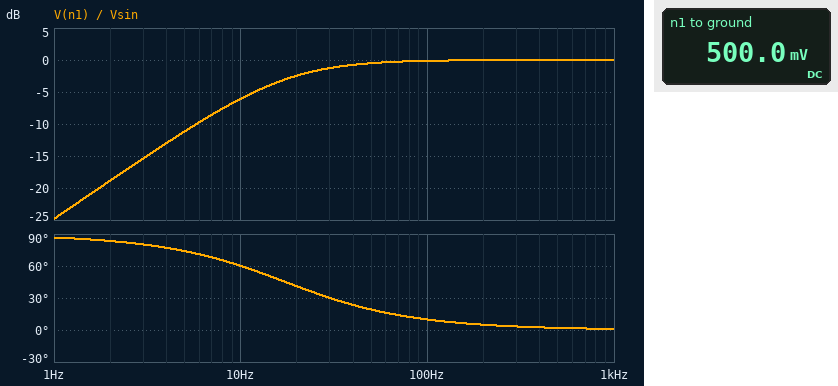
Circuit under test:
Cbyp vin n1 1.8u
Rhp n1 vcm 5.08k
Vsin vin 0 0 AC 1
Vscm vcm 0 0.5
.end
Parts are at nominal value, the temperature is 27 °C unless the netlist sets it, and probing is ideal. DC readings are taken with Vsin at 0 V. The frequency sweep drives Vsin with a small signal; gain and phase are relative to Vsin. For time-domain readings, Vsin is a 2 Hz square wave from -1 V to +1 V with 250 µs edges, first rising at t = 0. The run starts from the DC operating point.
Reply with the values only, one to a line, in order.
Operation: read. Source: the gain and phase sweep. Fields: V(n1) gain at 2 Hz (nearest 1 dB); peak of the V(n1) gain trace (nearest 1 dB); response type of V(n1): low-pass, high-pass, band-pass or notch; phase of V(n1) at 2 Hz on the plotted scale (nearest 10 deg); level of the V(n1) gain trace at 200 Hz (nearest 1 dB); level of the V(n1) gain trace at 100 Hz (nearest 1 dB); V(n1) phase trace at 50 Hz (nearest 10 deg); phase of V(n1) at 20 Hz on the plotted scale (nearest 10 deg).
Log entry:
-19 dB
0 dB
high-pass
80 deg
0 dB
0 dB
20 deg
40 deg
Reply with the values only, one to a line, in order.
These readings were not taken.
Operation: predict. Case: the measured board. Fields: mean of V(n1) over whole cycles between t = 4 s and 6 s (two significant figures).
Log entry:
500 mV
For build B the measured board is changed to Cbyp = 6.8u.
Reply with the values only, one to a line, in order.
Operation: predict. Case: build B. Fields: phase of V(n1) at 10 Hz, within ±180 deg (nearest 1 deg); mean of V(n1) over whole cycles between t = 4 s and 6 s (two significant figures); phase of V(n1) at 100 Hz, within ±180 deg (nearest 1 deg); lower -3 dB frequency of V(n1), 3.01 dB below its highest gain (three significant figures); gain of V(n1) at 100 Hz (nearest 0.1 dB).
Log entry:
25 deg
500 mV
3 deg
4.61 Hz
0 dB
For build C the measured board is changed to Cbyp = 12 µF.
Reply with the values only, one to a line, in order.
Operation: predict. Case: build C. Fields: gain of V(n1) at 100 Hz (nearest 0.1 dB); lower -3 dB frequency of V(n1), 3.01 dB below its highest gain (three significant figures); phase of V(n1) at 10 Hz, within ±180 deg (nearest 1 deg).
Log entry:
0 dB
2.61 Hz
15 deg
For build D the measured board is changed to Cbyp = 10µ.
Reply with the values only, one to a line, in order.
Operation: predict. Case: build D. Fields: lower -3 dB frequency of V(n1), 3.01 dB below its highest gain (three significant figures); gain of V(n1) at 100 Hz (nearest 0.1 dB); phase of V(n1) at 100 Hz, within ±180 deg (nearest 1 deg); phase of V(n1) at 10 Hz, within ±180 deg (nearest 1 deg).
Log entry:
3.13 Hz
0 dB
2 deg
17 deg
